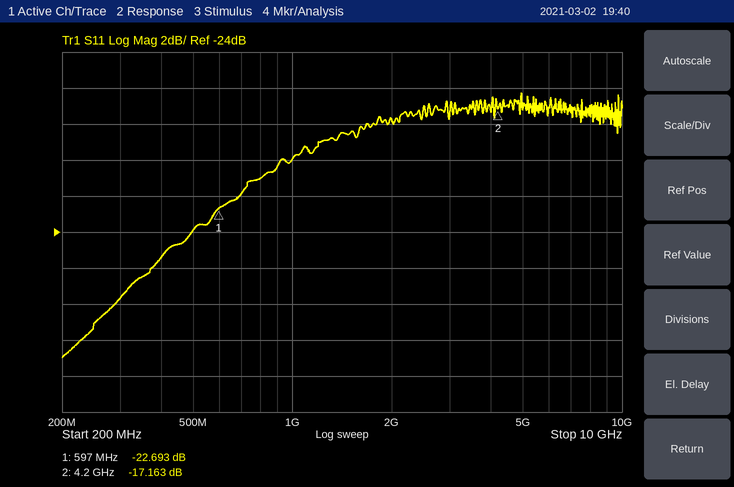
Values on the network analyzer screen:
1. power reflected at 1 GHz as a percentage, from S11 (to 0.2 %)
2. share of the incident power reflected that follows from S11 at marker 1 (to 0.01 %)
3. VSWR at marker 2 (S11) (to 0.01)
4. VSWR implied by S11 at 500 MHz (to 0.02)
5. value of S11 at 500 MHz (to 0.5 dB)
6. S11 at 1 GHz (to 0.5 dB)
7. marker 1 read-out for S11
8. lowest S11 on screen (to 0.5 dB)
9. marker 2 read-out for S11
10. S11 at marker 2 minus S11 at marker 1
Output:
1.0 %
0.54 %
1.32
1.14
-24.0 dB
-20.0 dB
-22.693 dB
-31.0 dB
-17.163 dB
5.530 dB
